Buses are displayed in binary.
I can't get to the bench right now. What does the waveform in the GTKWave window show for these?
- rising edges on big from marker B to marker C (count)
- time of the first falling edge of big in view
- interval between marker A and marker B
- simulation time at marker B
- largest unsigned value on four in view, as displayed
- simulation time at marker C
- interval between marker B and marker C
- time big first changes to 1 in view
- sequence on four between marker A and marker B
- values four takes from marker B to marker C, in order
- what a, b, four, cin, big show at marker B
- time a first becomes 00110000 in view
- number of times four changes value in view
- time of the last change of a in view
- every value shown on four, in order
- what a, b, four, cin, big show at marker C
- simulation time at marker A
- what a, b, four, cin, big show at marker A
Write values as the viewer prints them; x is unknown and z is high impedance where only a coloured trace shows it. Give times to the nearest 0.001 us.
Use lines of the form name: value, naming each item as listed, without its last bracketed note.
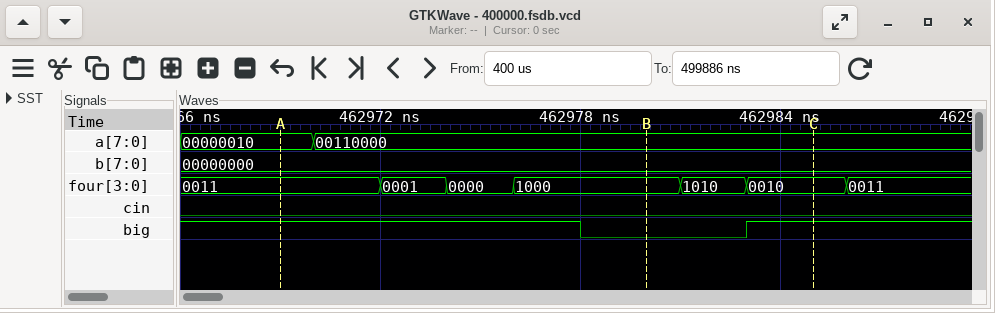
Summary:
rising edges on big from marker B to marker C: 1
time of the first falling edge of big in view: 462.978 us
interval between marker A and marker B: 0.011 us
simulation time at marker B: 462.98 us
largest unsigned value on four in view, as displayed: 1010
simulation time at marker C: 462.985 us
interval between marker B and marker C: 0.005 us
time big first changes to 1 in view: 462.983 us
sequence on four between marker A and marker B: 0011, 0001, 0000, 1000
values four takes from marker B to marker C, in order: 1000, 1010, 0010
what a, b, four, cin, big show at marker B: a=00110000, b=00000000, four=1000, cin=0, big=0
time a first becomes 00110000 in view: 462.97 us
number of times four changes value in view: 6
time of the last change of a in view: 462.97 us
every value shown on four, in order: 0011, 0001, 0000, 1000, 1010, 0010, 0011
what a, b, four, cin, big show at marker C: a=00110000, b=00000000, four=0010, cin=0, big=1
simulation time at marker A: 462.969 us
what a, b, four, cin, big show at marker A: a=00000010, b=00000000, four=0011, cin=0, big=1
